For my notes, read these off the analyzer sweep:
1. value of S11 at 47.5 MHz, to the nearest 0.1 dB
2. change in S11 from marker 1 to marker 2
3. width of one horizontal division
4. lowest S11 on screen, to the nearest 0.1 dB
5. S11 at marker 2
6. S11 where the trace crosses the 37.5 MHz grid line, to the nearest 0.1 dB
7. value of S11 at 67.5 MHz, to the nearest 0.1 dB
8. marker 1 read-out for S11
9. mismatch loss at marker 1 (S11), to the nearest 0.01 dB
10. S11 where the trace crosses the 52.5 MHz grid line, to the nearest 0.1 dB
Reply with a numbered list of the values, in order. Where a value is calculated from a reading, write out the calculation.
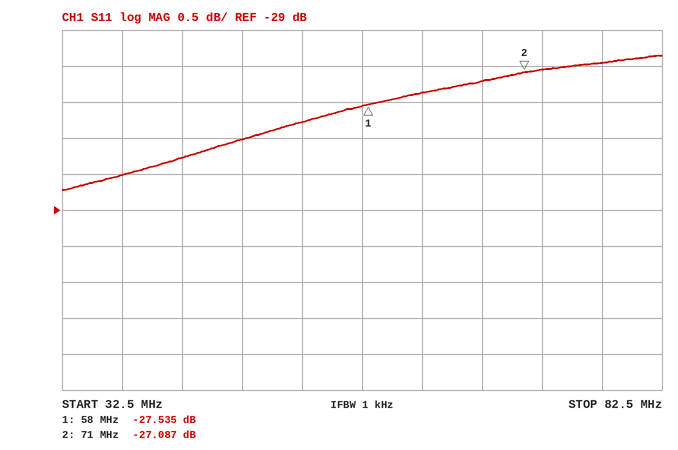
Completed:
1. -28.0 dB
2. -27.087 − (-27.535) = 0.448 dB
3. 5 MHz
4. -28.7 dB
5. -27.087 dB
6. -28.5 dB
7. -27.2 dB
8. -27.535 dB
9. −10 log10(1 − 10^(-27.535/10)) ≈ 0.01 dB
10. -27.8 dB
